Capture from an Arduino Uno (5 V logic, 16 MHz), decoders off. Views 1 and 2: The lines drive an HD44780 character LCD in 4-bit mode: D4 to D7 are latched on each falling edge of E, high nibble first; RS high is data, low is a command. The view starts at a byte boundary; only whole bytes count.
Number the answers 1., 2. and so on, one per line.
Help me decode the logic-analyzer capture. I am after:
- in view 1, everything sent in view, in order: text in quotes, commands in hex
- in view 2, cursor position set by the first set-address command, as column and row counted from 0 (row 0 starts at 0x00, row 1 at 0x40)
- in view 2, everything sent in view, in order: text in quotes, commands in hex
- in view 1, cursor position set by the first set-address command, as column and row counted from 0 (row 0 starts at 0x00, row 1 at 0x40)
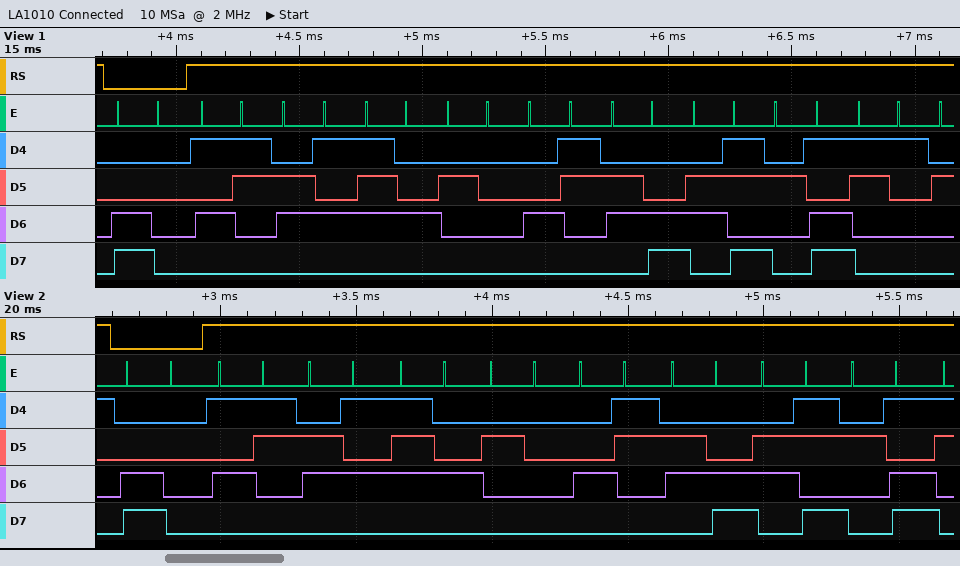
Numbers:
1. 0xC0 "Set Clk-1"
2. column 0, row 1
3. 0xC0 "Set Clk-"
4. column 0, row 1
